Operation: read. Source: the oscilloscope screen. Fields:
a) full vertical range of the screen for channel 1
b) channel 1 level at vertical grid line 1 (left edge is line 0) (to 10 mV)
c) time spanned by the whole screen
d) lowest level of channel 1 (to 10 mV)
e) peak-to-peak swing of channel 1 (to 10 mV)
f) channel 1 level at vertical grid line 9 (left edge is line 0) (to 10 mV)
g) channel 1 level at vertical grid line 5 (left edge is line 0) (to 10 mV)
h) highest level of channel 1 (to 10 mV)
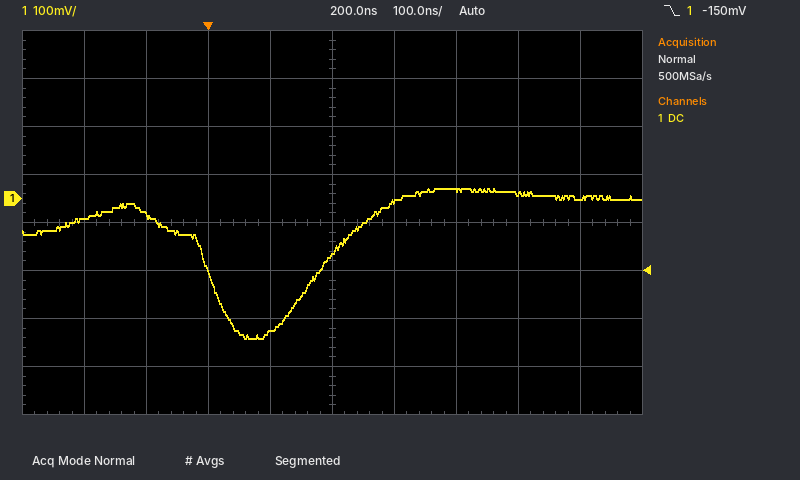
800 mV
-40 mV
1 µs
-290 mV
310 mV
0 mV
-120 mV
20 mV
